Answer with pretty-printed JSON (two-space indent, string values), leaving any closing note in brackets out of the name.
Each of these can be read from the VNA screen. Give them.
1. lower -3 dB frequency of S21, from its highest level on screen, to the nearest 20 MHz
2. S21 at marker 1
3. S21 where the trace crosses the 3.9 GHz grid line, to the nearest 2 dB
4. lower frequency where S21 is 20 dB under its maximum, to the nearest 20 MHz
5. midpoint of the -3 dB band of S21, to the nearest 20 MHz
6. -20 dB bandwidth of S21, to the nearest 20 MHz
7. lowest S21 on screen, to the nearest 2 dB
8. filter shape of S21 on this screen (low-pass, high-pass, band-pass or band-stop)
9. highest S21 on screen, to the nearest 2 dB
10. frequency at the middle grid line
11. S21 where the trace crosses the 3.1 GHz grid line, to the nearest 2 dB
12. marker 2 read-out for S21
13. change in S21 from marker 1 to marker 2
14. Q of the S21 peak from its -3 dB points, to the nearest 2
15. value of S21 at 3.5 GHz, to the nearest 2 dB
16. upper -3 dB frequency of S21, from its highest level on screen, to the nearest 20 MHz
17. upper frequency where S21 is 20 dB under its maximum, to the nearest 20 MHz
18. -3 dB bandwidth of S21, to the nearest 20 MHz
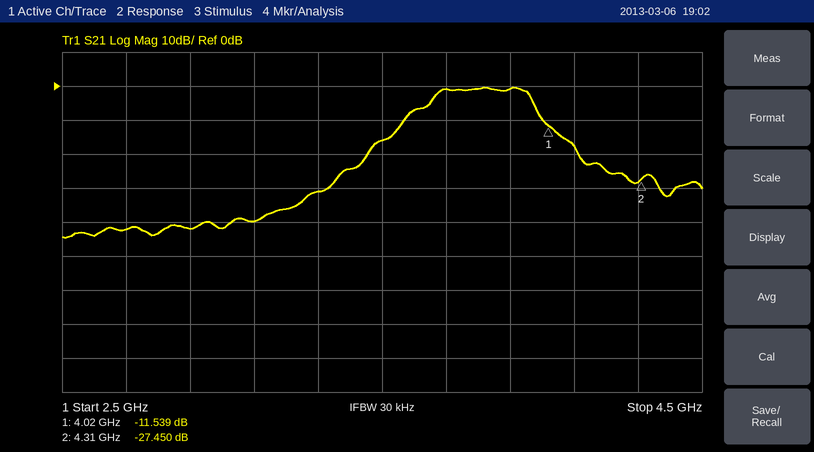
{
  "lower -3 dB frequency of S21, from its highest level on screen, to the nearest 20 MHz": "3.66 GHz",
  "S21 at marker 1": "-11.539 dB",
  "S21 where the trace crosses the 3.9 GHz grid line, to the nearest 2 dB": "0 dB",
  "lower frequency where S21 is 20 dB under its maximum, to the nearest 20 MHz": "3.46 GHz",
  "midpoint of the -3 dB band of S21, to the nearest 20 MHz": "3.82 GHz",
  "-20 dB bandwidth of S21, to the nearest 20 MHz": "660 MHz",
  "lowest S21 on screen, to the nearest 2 dB": "-44 dB",
  "filter shape of S21 on this screen": "band-pass",
  "highest S21 on screen, to the nearest 2 dB": "0 dB",
  "frequency at the middle grid line": "3.5 GHz",
  "S21 where the trace crosses the 3.1 GHz grid line, to the nearest 2 dB": "-40 dB",
  "marker 2 read-out for S21": "-27.450 dB",
  "change in S21 from marker 1 to marker 2": "-15.911 dB",
  "Q of the S21 peak from its -3 dB points, to the nearest 2": "12",
  "value of S21 at 3.5 GHz, to the nearest 2 dB": "-16 dB",
  "upper -3 dB frequency of S21, from its highest level on screen, to the nearest 20 MHz": "3.96 GHz",
  "upper frequency where S21 is 20 dB under its maximum, to the nearest 20 MHz": "4.12 GHz",
  "-3 dB bandwidth of S21, to the nearest 20 MHz": "300 MHz"
}
